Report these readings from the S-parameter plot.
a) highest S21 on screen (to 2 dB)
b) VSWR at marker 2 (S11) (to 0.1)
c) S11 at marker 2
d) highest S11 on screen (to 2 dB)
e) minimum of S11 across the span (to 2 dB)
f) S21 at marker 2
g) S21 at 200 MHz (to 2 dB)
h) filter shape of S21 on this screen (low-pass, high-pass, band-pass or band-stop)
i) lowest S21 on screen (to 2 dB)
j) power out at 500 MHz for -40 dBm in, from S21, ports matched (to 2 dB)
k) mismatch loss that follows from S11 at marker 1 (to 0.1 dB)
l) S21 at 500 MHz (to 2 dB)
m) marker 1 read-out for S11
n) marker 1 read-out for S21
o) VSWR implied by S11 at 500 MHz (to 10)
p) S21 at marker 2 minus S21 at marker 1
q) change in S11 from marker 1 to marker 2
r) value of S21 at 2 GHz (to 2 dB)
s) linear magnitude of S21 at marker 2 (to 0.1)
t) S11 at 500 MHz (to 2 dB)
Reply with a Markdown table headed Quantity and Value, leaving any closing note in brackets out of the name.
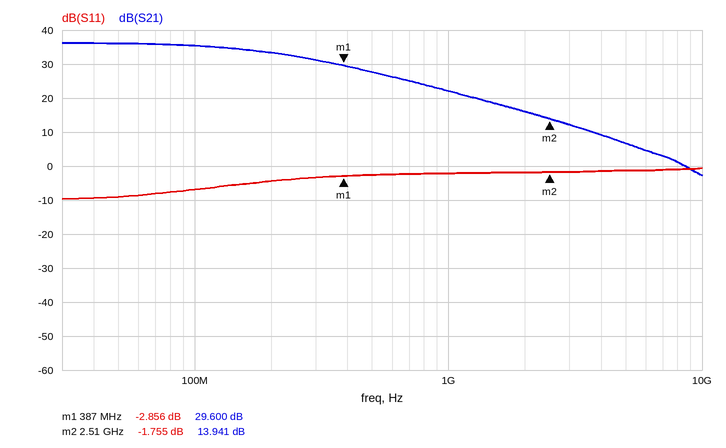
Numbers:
| Quantity | Value |
|---|---|
| highest S21 on screen | 36 dB |
| VSWR at marker 2 (S11) | 9.9 |
| S11 at marker 2 | -1.755 dB |
| highest S11 on screen | 0 dB |
| minimum of S11 across the span | -10 dB |
| S21 at marker 2 | 13.941 dB |
| S21 at 200 MHz | 34 dB |
| filter shape of S21 on this screen | low-pass |
| lowest S21 on screen | -2 dB |
| power out at 500 MHz for -40 dBm in, from S21, ports matched | -12 dBm |
| mismatch loss that follows from S11 at marker 1 | 3.2 dB |
| S21 at 500 MHz | 28 dB |
| marker 1 read-out for S11 | -2.856 dB |
| marker 1 read-out for S21 | 29.600 dB |
| VSWR implied by S11 at 500 MHz | 10 |
| S21 at marker 2 minus S21 at marker 1 | -15.659 dB |
| change in S11 from marker 1 to marker 2 | 1.101 dB |
| value of S21 at 2 GHz | 16 dB |
| linear magnitude of S21 at marker 2 | 5.0 |
| S11 at 500 MHz | -2 dB |
